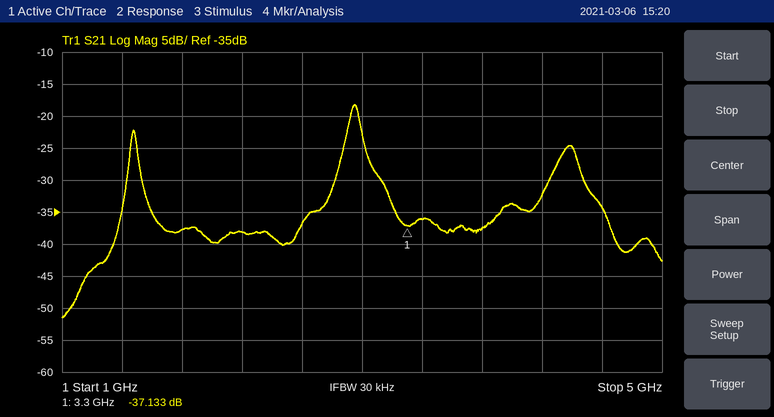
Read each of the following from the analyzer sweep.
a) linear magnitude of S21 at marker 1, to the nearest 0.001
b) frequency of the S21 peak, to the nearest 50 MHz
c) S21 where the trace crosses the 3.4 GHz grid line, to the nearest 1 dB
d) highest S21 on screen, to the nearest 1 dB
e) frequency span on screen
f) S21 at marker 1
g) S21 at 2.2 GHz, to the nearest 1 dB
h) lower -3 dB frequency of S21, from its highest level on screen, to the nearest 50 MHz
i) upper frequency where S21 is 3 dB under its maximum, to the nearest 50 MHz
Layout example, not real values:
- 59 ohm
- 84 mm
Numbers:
- 0.014
- 2.95 GHz
- -36 dB
- -18 dB
- 4 GHz
- -37.133 dB
- -38 dB
- 2.90 GHz
- 3.00 GHz
